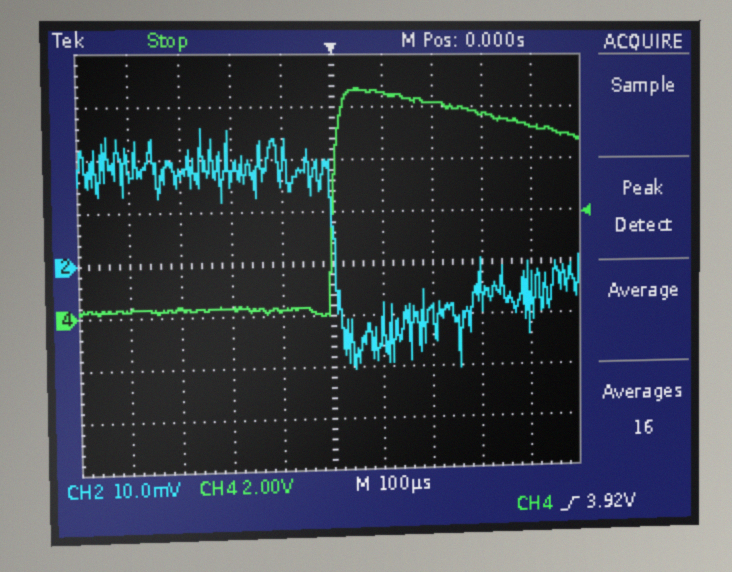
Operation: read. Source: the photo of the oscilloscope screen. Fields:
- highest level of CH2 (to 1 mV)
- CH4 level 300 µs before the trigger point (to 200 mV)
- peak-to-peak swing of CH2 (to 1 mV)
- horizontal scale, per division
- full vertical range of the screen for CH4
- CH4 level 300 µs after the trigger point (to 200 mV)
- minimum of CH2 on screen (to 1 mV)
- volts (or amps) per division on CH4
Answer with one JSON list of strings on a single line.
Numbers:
["26 mV", "400 mV", "46 mV", "100 µs", "16 V", "7.8 V", "-20 mV", "2 V"]
